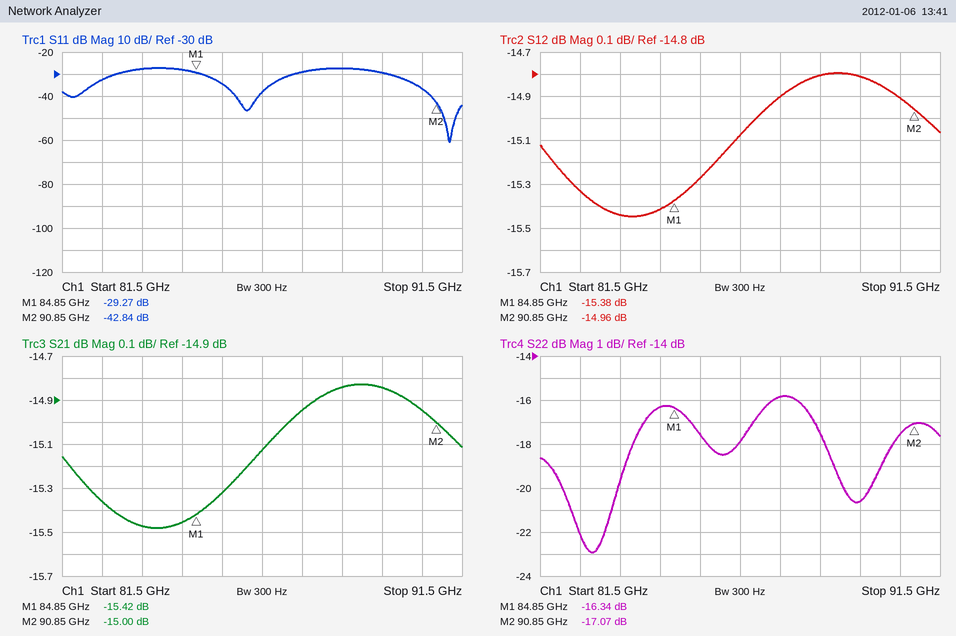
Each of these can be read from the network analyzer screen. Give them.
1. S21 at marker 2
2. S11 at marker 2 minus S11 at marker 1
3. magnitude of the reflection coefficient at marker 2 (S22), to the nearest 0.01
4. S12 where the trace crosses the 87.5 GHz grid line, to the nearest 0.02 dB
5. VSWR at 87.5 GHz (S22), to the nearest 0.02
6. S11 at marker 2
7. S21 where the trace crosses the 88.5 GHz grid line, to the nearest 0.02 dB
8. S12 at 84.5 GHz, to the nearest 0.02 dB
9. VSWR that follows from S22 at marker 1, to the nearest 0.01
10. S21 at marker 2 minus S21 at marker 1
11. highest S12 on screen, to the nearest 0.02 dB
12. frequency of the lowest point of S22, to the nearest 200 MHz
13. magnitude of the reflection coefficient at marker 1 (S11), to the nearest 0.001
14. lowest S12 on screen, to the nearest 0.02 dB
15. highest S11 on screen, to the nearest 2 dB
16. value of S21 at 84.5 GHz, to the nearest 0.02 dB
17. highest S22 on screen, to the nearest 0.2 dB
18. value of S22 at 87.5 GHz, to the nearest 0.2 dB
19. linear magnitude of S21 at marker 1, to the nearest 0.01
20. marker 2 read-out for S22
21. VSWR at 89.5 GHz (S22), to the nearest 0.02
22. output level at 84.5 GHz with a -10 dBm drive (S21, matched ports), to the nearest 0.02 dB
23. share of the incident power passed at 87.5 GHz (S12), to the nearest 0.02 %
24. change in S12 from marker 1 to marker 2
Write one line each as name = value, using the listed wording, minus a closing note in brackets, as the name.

S21 at marker 2 = -15.00 dB
S11 at marker 2 minus S11 at marker 1 = -13.57 dB
magnitude of the reflection coefficient at marker 2 (S22), to the nearest 0.01 = 0.14
S12 where the trace crosses the 87.5 GHz grid line, to the nearest 0.02 dB = -14.90 dB
VSWR at 87.5 GHz (S22), to the nearest 0.02 = 1.38
S11 at marker 2 = -42.84 dB
S21 where the trace crosses the 88.5 GHz grid line, to the nearest 0.02 dB = -14.84 dB
S12 at 84.5 GHz, to the nearest 0.02 dB = -15.42 dB
VSWR that follows from S22 at marker 1, to the nearest 0.01 = 1.36
S21 at marker 2 minus S21 at marker 1 = 0.42 dB
highest S12 on screen, to the nearest 0.02 dB = -14.80 dB
frequency of the lowest point of S22, to the nearest 200 MHz = 82.8 GHz
magnitude of the reflection coefficient at marker 1 (S11), to the nearest 0.001 = 0.034
lowest S12 on screen, to the nearest 0.02 dB = -15.44 dB
highest S11 on screen, to the nearest 2 dB = -28 dB
value of S21 at 84.5 GHz, to the nearest 0.02 dB = -15.46 dB
highest S22 on screen, to the nearest 0.2 dB = -15.8 dB
value of S22 at 87.5 GHz, to the nearest 0.2 dB = -15.8 dB
linear magnitude of S21 at marker 1, to the nearest 0.01 = 0.17
marker 2 read-out for S22 = -17.07 dB
VSWR at 89.5 GHz (S22), to the nearest 0.02 = 1.20
output level at 84.5 GHz with a -10 dBm drive (S21, matched ports), to the nearest 0.02 dB = -25.46 dBm
share of the incident power passed at 87.5 GHz (S12), to the nearest 0.02 % = 3.24 %
change in S12 from marker 1 to marker 2 = 0.42 dB
